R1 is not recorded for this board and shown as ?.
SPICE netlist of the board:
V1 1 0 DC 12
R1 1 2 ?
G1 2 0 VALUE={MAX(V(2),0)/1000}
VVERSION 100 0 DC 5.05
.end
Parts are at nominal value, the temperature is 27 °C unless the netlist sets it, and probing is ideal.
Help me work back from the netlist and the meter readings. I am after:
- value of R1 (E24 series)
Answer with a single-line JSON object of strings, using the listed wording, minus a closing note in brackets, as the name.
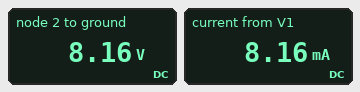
{"value of R1": "470 Ω"}
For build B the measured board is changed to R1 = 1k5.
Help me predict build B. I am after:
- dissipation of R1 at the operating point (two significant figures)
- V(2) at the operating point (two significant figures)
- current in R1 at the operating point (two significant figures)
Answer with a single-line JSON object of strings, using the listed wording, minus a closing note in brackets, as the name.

{"dissipation of R1 at the operating point": "35 mW", "V(2) at the operating point": "4.8 V", "current in R1 at the operating point": "4.8 mA"}
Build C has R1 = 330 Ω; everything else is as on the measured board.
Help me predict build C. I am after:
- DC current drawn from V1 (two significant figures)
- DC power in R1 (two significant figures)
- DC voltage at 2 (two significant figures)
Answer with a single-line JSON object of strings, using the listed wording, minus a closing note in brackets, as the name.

{"DC current drawn from V1": "9.0 mA", "DC power in R1": "27 mW", "DC voltage at 2": "9.0 V"}
